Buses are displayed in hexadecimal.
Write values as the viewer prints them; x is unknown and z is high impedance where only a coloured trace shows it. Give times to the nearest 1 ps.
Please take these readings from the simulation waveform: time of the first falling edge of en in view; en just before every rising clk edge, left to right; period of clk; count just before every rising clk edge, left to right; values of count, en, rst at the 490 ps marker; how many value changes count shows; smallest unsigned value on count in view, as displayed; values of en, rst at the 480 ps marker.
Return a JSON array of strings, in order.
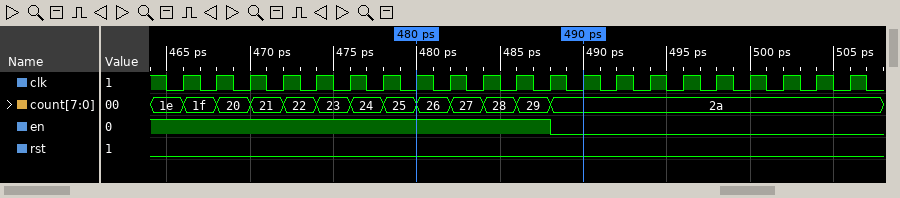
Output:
["488 ps", "1 1 1 1 1 1 1 1 1 1 1 1 0 0 0 0 0 0 0 0 0", "2 ps", "1e, 1f, 20, 21, 22, 23, 24, 25, 26, 27, 28, 29, 2a, 2a, 2a, 2a, 2a, 2a, 2a, 2a, 2a", "count=2a, en=0, rst=0", "12", "1e", "en=1, rst=0"]
